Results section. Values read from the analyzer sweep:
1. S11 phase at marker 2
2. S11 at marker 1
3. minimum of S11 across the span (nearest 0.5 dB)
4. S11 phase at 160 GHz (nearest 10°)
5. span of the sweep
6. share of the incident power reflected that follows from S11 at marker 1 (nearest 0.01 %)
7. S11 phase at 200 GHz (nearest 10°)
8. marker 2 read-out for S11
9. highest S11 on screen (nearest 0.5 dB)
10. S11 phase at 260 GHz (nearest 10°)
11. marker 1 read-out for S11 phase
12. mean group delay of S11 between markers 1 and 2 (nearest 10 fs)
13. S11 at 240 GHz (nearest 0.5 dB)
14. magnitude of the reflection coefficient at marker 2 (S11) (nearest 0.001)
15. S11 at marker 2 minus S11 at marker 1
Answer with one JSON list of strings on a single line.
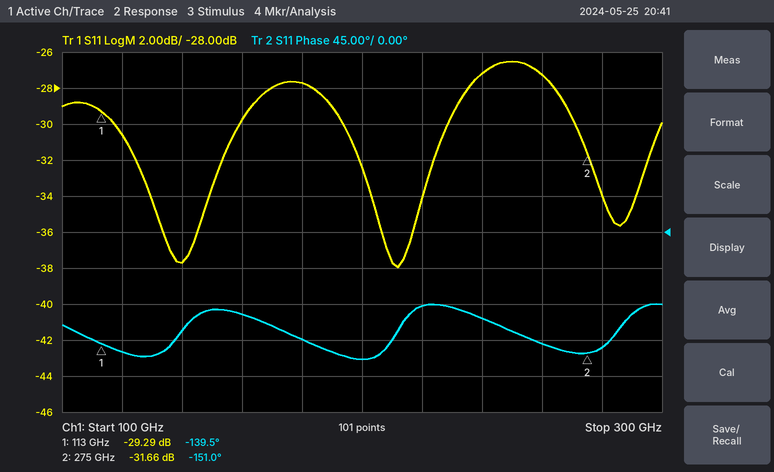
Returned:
["-151.0°", "-29.29 dB", "-38.0 dB", "-100°", "200 GHz", "0.12 %", "-160°", "-31.66 dB", "-26.5 dB", "-140°", "-139.5°", "200 fs", "-27.0 dB", "0.026", "-2.37 dB"]
